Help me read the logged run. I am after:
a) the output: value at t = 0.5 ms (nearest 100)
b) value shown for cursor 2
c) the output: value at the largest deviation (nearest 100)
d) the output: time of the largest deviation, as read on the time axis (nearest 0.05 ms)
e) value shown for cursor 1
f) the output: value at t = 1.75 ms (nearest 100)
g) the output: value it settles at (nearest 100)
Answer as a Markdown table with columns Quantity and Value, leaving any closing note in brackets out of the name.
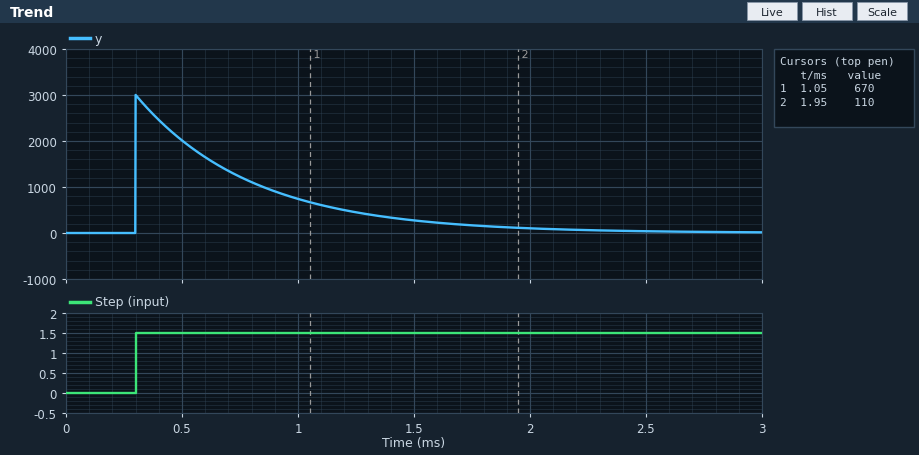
| Quantity | Value |
|---|---|
| the output: value at t = 0.5 ms | 2000 |
| value shown for cursor 2 | 110 |
| the output: value at the largest deviation | 3000 |
| the output: time of the largest deviation, as read on the time axis | 0.30 ms |
| value shown for cursor 1 | 670 |
| the output: value at t = 1.75 ms | 200 |
| the output: value it settles at | 0 |
